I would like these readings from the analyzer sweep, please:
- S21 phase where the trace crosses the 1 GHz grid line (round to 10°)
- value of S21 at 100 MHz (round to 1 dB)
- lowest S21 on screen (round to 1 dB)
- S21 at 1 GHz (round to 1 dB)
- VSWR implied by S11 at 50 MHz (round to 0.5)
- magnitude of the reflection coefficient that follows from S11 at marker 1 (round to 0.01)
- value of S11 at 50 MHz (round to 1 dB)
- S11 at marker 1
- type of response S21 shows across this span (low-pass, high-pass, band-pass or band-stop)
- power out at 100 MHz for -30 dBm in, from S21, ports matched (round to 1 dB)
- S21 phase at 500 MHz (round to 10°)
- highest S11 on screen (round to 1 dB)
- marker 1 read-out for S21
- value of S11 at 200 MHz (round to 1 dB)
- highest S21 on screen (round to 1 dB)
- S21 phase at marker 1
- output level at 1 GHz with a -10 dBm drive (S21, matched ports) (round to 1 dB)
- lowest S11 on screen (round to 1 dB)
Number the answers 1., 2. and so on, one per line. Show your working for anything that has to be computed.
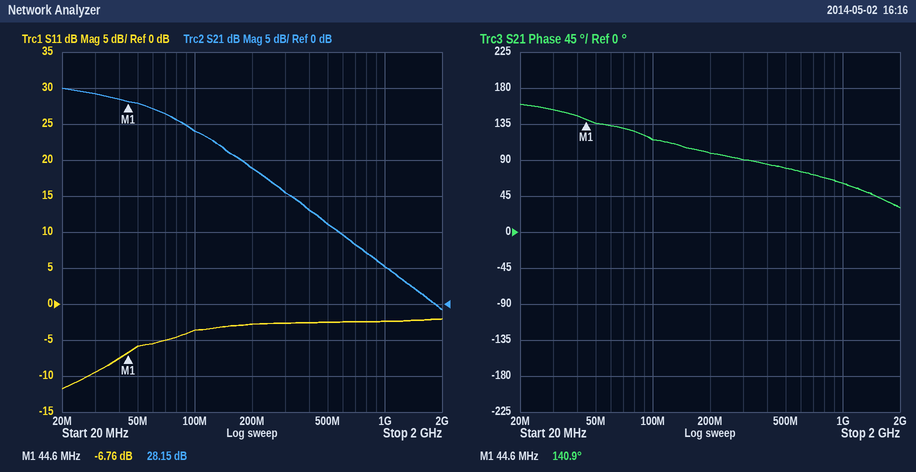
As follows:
1. 60°
2. 24 dB
3. -1 dB
4. 5 dB
5. |Γ| = 10^(-6/20) = 0.5012; VSWR = (1 + 0.5012)/(1 − 0.5012) ≈ 3.0
6. 10^(-6.76/20) ≈ 0.46
7. -6 dB
8. -6.76 dB
9. low-pass
10. -30 dBm + (24 dB) = -6 dBm
11. 80°
12. -2 dB
13. 28.15 dB
14. -3 dB
15. 30 dB
16. 140.9°
17. -10 dBm + (5 dB) = -5 dBm
18. -12 dB
